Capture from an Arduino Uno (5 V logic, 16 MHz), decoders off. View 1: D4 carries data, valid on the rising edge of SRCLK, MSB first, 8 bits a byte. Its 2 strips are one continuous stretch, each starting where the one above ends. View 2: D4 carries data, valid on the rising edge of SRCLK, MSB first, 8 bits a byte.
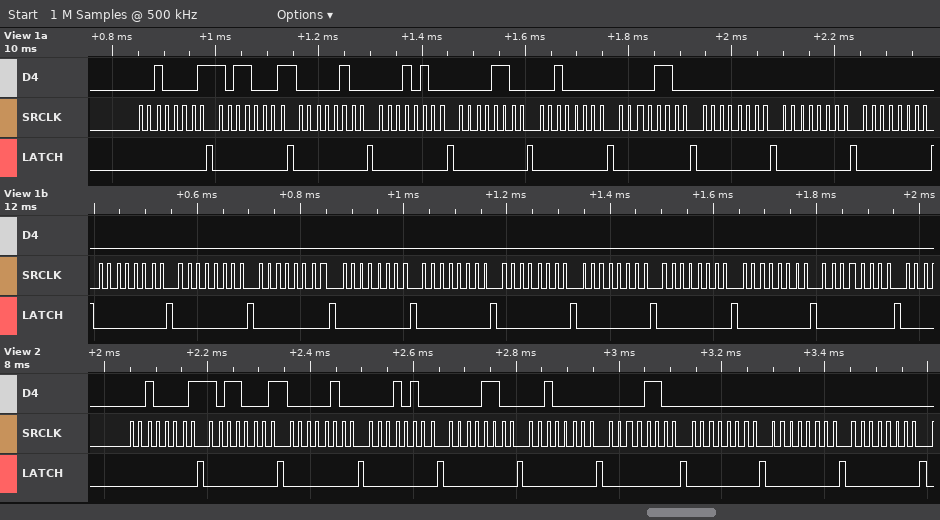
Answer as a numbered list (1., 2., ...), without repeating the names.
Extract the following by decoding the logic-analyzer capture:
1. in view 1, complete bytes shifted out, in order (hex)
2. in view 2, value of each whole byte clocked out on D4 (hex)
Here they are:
1. 0x21 0xB1 0x04 0x14 0x0C 0x20 0x0C 0x00 0x00 0x00 0x00 0x00 0x00 0x00 0x00 0x00 0x00 0x00 0x00 0x00
2. 0x21 0xB1 0x04 0x14 0x0C 0x20 0x0C 0x00 0x00 0x00
